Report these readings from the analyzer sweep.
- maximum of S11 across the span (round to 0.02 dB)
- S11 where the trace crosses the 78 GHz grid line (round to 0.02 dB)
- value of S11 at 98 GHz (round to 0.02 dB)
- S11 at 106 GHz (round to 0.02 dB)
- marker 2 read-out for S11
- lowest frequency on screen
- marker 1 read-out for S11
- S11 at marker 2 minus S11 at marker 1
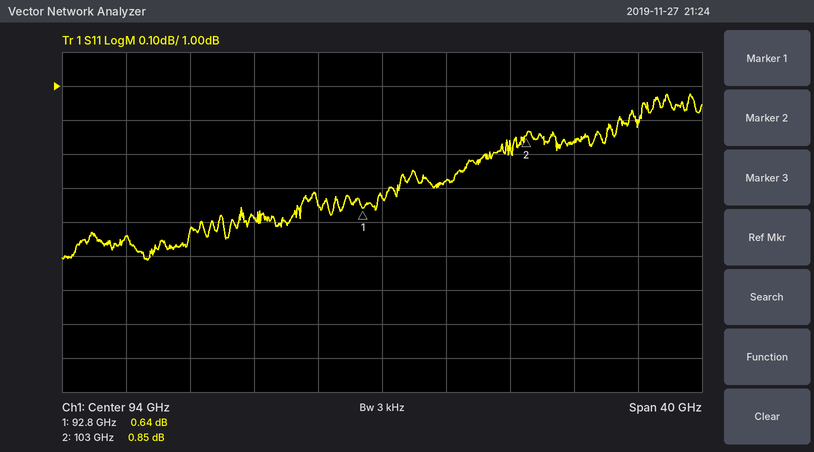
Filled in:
0.98 dB
0.56 dB
0.72 dB
0.84 dB
0.85 dB
74 GHz
0.64 dB
0.21 dB
